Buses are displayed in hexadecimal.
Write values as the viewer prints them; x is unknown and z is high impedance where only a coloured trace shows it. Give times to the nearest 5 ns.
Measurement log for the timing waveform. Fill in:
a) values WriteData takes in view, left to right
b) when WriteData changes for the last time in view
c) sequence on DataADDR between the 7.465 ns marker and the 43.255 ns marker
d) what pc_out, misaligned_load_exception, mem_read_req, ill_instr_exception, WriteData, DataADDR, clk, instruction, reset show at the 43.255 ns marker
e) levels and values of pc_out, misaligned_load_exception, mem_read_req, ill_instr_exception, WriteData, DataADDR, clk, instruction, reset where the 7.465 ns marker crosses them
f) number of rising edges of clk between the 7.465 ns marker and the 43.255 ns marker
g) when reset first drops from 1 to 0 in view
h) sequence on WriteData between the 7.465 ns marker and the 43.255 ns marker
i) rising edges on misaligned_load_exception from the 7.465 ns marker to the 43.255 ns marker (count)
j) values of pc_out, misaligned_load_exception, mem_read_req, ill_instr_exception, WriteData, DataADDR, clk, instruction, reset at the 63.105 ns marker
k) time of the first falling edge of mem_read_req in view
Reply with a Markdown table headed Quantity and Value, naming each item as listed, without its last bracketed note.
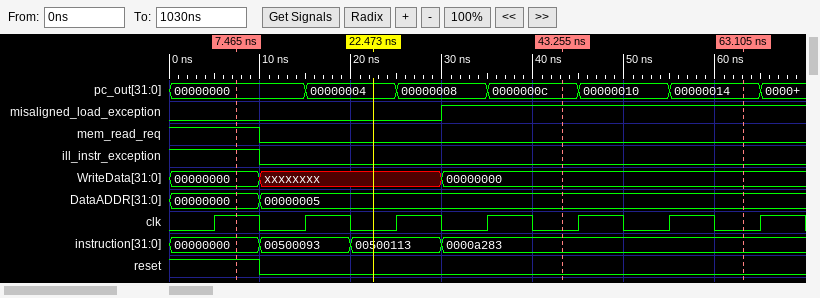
| Quantity | Value |
|---|---|
| values WriteData takes in view, left to right | 00000000, xxxxxxxx, 00000000 |
| when WriteData changes for the last time in view | 30 ns |
| sequence on DataADDR between the 7.465 ns marker and the 43.255 ns marker | 00000000, 00000005 |
| what pc_out, misaligned_load_exception, mem_read_req, ill_instr_exception, WriteData, DataADDR, clk, instruction, reset show at the 43.255 ns marker | pc_out=0000000c, misaligned_load_exception=1, mem_read_req=0, ill_instr_exception=0, WriteData=00000000, DataADDR=00000005, clk=0, instruction=0000a283, reset=0 |
| levels and values of pc_out, misaligned_load_exception, mem_read_req, ill_instr_exception, WriteData, DataADDR, clk, instruction, reset where the 7.465 ns marker crosses them | pc_out=00000000, misaligned_load_exception=0, mem_read_req=1, ill_instr_exception=1, WriteData=00000000, DataADDR=00000000, clk=1, instruction=00000000, reset=1 |
| number of rising edges of clk between the 7.465 ns marker and the 43.255 ns marker | 3 |
| when reset first drops from 1 to 0 in view | 10 ns |
| sequence on WriteData between the 7.465 ns marker and the 43.255 ns marker | 00000000, xxxxxxxx, 00000000 |
| rising edges on misaligned_load_exception from the 7.465 ns marker to the 43.255 ns marker | 1 |
| values of pc_out, misaligned_load_exception, mem_read_req, ill_instr_exception, WriteData, DataADDR, clk, instruction, reset at the 63.105 ns marker | pc_out=00000014, misaligned_load_exception=1, mem_read_req=0, ill_instr_exception=0, WriteData=00000000, DataADDR=00000005, clk=0, instruction=0000a283, reset=0 |
| time of the first falling edge of mem_read_req in view | 10 ns |
